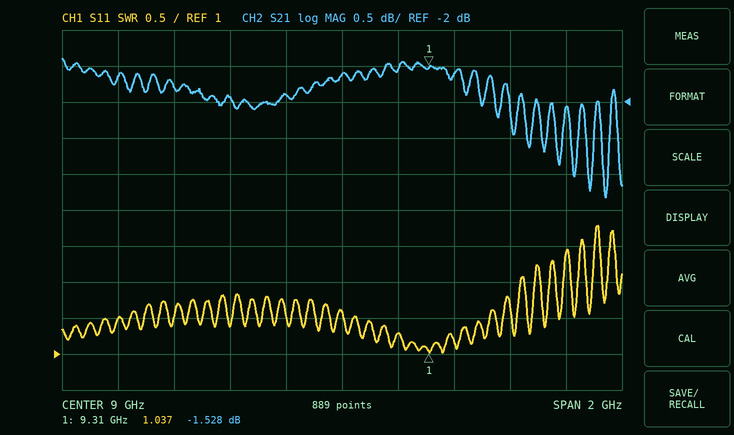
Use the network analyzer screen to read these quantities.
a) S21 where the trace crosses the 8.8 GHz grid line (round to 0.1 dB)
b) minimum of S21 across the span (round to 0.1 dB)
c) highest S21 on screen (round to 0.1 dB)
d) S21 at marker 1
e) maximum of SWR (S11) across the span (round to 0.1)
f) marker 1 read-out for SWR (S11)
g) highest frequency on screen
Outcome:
-1.9 dB
-3.3 dB
-1.4 dB
-1.528 dB
2.8
1.037
10 GHz
